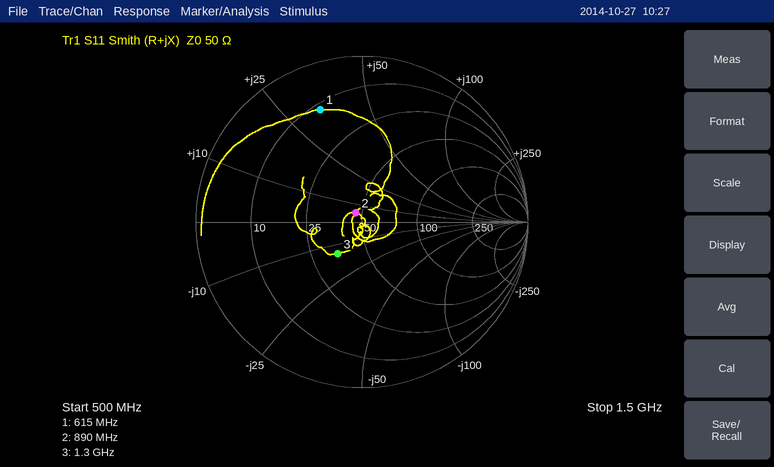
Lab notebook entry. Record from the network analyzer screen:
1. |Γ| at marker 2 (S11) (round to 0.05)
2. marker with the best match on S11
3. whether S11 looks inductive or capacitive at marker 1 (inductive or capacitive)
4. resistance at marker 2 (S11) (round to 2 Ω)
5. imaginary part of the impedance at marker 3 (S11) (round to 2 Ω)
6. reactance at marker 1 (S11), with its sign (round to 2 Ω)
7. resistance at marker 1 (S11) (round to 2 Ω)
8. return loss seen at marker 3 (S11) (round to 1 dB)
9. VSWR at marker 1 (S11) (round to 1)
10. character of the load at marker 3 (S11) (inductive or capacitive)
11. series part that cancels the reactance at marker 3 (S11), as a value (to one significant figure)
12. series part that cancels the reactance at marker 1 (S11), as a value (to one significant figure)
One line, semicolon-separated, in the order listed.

0.05; marker 2; inductive; 46 Ω; -14 Ω; +34 Ω; 12 Ω; 12 dB; 6; capacitive; 2 nH; 8 pF
